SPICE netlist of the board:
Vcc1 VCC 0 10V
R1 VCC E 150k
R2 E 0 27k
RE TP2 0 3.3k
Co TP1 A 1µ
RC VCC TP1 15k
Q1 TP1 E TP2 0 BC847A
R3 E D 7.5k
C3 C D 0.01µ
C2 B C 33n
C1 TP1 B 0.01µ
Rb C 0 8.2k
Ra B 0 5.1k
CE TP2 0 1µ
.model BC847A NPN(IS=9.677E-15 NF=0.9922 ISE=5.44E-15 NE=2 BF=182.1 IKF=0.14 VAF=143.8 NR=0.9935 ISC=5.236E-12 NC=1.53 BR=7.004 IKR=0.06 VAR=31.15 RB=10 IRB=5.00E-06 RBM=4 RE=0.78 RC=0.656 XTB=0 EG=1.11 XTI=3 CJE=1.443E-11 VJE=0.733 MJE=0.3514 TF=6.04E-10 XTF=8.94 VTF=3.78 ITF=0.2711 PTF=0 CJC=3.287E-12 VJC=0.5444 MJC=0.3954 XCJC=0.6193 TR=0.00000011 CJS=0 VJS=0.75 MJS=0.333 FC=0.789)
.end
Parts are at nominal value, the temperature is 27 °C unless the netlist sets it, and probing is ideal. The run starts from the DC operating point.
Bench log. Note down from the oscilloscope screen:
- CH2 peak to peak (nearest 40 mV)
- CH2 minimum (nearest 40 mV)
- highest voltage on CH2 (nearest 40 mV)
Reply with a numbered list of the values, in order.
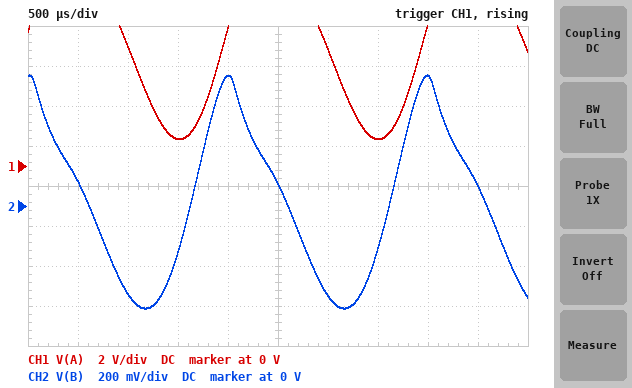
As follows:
1. 1.16 V
2. -520 mV
3. 640 mV
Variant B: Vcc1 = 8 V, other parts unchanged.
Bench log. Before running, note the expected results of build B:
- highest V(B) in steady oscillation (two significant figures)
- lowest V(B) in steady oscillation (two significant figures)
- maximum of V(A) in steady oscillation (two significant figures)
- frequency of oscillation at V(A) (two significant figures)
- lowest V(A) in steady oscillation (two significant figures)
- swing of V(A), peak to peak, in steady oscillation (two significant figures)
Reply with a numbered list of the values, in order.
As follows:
1. 370 mV
2. -310 mV
3. 7.6 V
4. 510 Hz
5. 2.5 V
6. 5.1 V
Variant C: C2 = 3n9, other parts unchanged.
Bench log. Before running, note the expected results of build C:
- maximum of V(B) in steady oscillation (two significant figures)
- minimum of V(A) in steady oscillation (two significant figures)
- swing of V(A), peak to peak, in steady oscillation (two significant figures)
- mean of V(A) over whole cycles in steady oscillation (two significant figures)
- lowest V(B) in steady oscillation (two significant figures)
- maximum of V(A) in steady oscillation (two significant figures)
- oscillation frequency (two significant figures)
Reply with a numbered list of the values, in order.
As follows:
1. 800 mV
2. 3.3 V
3. 5.2 V
4. 6.0 V
5. -700 mV
6. 8.5 V
7. 950 Hz
